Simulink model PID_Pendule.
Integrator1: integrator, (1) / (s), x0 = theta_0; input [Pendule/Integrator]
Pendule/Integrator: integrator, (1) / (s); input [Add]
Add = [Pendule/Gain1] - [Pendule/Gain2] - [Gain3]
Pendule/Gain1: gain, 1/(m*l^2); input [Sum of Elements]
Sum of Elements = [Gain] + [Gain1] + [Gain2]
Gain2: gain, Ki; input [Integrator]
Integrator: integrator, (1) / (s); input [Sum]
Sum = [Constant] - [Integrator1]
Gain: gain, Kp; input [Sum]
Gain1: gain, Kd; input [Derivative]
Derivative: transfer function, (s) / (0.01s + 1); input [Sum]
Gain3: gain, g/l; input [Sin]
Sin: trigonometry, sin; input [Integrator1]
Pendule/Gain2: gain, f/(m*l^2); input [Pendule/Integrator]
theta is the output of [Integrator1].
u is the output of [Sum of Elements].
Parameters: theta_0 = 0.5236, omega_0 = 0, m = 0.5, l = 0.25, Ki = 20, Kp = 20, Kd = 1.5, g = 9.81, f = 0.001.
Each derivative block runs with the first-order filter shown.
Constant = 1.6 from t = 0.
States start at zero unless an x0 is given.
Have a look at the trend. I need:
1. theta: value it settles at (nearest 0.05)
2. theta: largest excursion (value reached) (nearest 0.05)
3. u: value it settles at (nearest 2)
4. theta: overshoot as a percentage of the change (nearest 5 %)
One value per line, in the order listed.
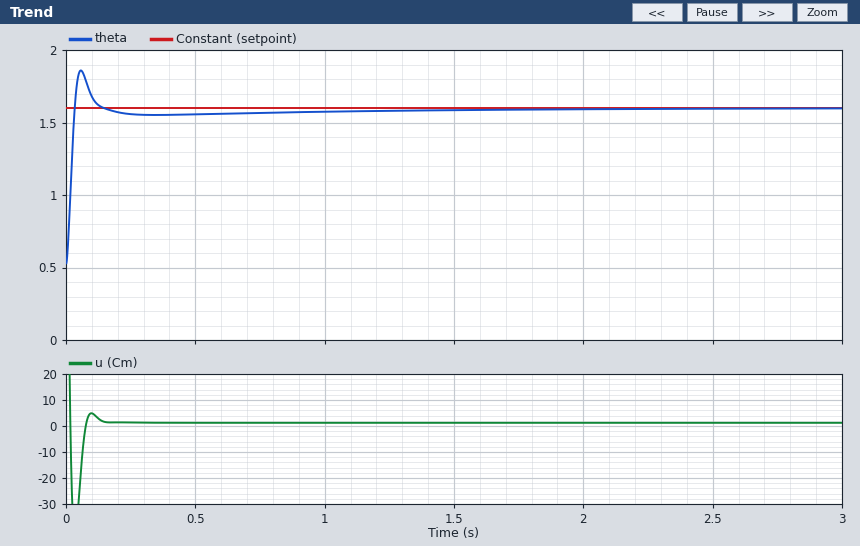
1.60
1.85
2
25 %
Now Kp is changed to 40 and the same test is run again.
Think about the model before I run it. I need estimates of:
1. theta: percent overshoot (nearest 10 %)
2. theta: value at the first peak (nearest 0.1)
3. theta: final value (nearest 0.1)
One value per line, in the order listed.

40 %
2.0
1.6
